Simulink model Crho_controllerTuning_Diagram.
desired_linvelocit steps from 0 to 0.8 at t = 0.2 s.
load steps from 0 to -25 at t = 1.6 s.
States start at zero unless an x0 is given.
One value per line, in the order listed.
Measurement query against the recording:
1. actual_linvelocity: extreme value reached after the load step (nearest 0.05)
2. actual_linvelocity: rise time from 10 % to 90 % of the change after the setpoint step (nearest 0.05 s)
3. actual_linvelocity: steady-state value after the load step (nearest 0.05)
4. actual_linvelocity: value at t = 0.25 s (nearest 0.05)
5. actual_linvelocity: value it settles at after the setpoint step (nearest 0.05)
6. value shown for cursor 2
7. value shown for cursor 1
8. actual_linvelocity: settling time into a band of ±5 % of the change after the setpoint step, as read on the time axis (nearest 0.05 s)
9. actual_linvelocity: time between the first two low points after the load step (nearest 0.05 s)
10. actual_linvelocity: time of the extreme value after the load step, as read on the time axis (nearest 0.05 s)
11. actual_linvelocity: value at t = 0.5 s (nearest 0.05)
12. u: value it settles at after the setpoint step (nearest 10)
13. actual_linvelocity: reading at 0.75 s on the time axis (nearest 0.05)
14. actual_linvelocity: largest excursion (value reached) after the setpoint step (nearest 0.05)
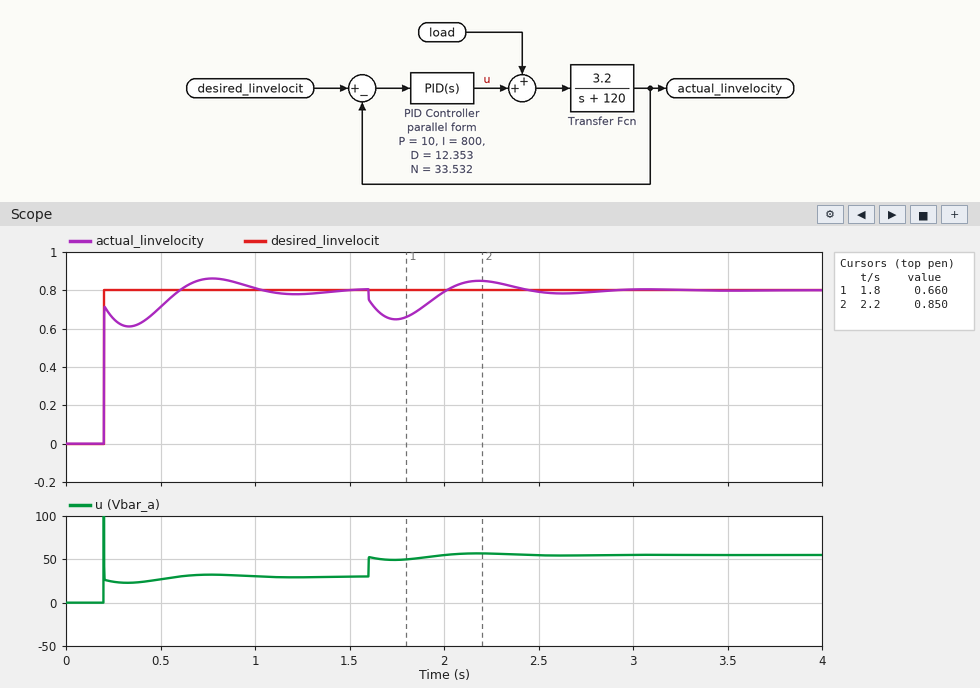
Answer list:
0.65
0.30 s
0.80
0.65
0.80
0.850
0.660
0.90 s
0.90 s
1.75 s
0.70
30
0.85
0.85
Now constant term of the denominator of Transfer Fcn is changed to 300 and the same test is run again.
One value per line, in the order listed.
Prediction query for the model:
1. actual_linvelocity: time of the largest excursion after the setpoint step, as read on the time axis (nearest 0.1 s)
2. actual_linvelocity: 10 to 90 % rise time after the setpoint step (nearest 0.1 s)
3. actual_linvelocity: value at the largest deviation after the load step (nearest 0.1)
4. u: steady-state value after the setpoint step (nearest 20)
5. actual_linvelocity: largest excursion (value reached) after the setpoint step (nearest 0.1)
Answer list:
0.9 s
0.4 s
0.7
80
0.8
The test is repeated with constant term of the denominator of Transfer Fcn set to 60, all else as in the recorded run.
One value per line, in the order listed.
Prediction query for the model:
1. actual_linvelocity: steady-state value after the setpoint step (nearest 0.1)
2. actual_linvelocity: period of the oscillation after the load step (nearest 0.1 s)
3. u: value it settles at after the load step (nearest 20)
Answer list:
0.8
0.8 s
40
